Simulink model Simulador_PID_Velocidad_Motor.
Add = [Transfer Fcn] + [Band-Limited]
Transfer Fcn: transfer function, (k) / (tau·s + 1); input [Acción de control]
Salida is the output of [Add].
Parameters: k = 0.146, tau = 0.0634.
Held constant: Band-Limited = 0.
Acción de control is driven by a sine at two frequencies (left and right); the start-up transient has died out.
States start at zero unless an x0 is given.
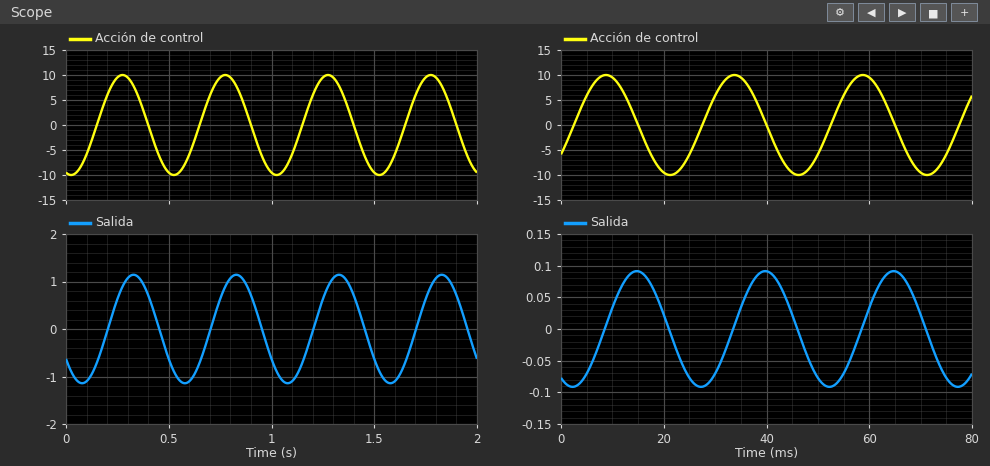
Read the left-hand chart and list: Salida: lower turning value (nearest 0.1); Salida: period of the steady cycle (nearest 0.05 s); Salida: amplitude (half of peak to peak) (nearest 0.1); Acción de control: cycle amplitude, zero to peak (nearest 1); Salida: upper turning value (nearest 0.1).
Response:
-1.1
0.50 s
1.1
10
1.1
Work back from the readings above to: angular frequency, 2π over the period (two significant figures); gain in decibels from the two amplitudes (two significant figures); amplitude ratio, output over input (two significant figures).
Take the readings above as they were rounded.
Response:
13 rad/s
-19 dB
0.11
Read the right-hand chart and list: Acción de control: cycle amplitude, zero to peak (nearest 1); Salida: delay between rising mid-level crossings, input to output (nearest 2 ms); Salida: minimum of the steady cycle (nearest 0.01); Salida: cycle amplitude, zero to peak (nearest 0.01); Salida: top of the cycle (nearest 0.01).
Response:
10
6 ms
-0.09
0.09
0.09
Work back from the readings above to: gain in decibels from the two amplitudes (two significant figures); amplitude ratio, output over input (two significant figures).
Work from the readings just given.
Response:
-41 dB
0.0090
